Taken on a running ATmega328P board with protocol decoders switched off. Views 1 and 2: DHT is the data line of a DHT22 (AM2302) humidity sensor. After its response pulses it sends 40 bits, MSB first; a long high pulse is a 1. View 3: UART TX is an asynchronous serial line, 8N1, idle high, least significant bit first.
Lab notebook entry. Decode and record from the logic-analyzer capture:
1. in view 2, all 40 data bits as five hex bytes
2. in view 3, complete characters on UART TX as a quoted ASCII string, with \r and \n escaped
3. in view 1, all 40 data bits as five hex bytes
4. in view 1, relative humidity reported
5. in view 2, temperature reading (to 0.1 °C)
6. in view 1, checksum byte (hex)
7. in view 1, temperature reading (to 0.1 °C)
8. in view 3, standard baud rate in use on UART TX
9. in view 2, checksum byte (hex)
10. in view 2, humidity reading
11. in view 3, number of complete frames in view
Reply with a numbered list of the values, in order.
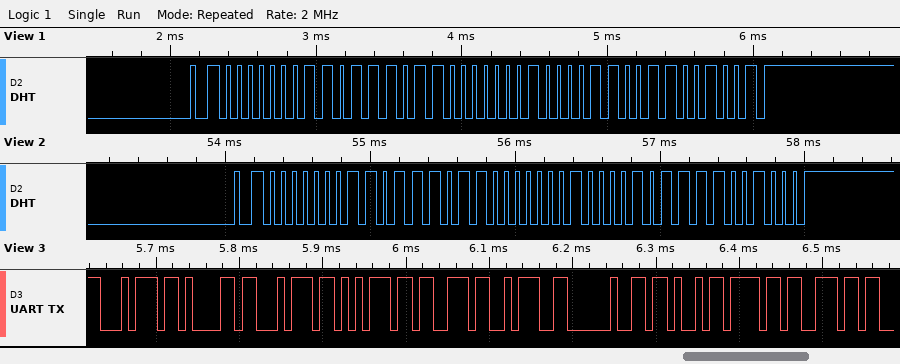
1. 01 BB 01 0B C8
2. "tatus: Kon"
3. 01 BB 01 0C C9
4. 44.3 %
5. 26.7 °C
6. 0xC9
7. 26.8 °C
8. 115200 baud
9. 0xC8
10. 44.3 %
11. 10
